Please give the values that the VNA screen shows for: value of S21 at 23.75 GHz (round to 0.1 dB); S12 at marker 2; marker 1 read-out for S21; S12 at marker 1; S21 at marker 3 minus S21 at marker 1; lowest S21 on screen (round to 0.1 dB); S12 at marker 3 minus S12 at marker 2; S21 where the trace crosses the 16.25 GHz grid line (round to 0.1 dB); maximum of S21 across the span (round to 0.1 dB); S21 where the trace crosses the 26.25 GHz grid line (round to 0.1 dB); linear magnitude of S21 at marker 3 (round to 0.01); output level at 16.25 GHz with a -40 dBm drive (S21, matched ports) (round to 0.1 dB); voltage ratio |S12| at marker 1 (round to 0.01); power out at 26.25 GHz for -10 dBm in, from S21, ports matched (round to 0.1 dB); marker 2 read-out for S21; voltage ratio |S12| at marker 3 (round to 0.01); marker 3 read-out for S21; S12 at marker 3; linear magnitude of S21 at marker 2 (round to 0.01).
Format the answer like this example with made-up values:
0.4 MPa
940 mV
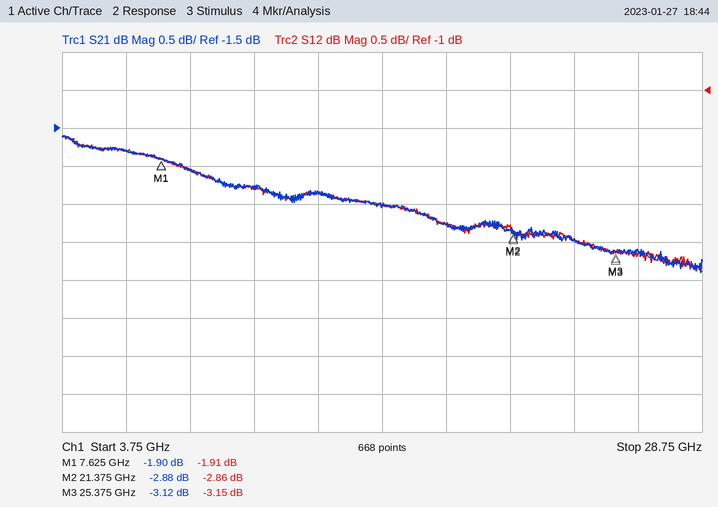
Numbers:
-3.0 dB
-2.86 dB
-1.90 dB
-1.91 dB
-1.22 dB
-3.4 dB
-0.29 dB
-2.5 dB
-1.6 dB
-3.1 dB
0.70
-42.5 dBm
0.80
-13.1 dBm
-2.88 dB
0.70
-3.12 dB
-3.15 dB
0.72
